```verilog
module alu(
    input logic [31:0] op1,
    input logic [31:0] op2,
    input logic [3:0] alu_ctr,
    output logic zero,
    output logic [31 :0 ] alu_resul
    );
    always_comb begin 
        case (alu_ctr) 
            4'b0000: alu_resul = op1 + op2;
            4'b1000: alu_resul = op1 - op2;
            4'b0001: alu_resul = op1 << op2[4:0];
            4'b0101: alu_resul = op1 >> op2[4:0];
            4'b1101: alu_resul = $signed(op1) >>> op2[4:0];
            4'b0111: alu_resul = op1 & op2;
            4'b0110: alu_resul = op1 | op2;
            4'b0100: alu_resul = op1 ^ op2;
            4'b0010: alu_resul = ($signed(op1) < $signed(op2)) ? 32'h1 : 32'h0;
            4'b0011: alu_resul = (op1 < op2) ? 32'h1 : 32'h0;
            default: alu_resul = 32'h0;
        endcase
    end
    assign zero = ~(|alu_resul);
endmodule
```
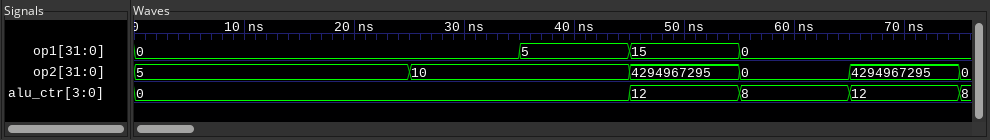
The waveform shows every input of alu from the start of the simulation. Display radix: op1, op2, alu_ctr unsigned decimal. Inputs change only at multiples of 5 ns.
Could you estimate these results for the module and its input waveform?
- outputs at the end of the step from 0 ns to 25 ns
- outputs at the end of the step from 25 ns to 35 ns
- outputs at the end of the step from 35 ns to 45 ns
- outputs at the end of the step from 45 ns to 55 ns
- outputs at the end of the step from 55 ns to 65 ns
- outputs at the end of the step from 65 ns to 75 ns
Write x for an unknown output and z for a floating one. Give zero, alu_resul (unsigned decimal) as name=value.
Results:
zero=0, alu_resul=5
zero=0, alu_resul=10
zero=0, alu_resul=15
zero=1, alu_resul=0
zero=1, alu_resul=0
zero=1, alu_resul=0
